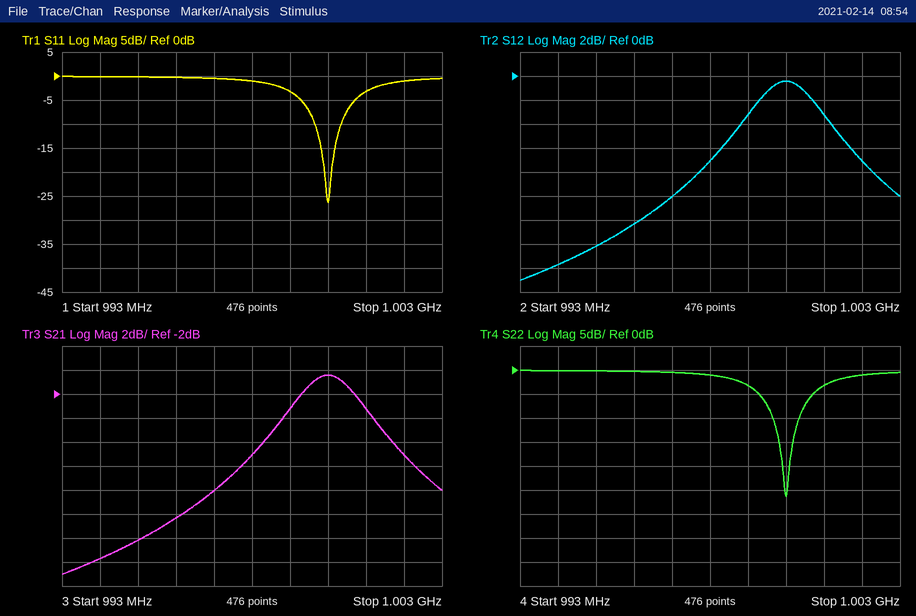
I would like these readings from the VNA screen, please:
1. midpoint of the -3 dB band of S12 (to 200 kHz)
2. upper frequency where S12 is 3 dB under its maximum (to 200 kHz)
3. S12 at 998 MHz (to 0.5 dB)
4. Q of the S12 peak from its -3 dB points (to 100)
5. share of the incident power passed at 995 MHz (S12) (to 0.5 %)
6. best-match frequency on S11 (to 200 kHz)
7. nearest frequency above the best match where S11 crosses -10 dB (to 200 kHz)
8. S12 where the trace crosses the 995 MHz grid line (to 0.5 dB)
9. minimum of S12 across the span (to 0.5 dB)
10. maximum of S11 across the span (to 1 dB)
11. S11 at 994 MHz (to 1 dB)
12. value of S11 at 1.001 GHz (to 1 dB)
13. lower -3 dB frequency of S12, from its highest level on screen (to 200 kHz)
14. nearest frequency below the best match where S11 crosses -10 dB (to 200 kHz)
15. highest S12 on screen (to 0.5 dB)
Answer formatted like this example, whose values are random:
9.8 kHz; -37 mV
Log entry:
1.0000 GHz; 1.0010 GHz; -7.0 dB; 500; 4.0 %; 1.0000 GHz; 1.0004 GHz; -14.0 dB; -17.0 dB; 0 dB; 0 dB; -3 dB; 999.0 MHz; 999.6 MHz; -0.5 dB
